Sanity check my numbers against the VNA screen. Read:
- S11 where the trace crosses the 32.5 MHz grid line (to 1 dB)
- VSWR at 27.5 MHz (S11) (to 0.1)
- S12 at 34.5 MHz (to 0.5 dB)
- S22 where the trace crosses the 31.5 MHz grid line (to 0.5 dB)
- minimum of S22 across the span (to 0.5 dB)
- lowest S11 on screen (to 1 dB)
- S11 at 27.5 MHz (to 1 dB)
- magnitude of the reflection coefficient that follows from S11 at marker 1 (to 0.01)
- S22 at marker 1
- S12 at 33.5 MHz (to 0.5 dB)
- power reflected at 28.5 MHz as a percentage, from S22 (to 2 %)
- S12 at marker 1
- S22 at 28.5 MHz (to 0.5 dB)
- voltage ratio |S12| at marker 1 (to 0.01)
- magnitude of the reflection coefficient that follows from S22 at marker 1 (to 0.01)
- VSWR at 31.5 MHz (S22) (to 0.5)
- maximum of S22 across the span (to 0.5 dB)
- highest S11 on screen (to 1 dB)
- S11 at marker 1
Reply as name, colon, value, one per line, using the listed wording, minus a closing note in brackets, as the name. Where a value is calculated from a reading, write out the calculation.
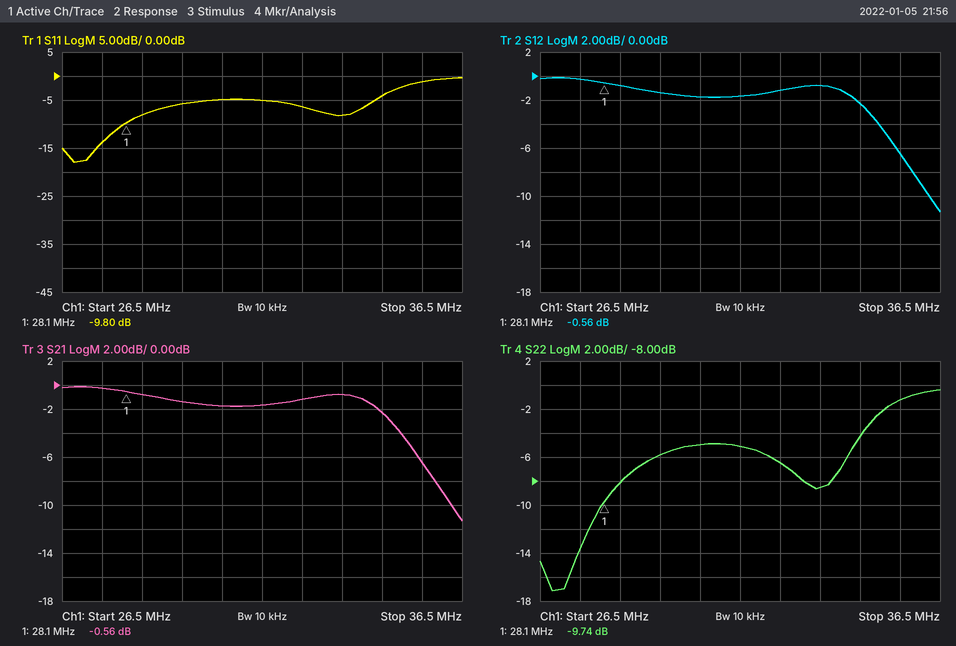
S11 where the trace crosses the 32.5 MHz grid line: -6 dB
VSWR at 27.5 MHz (S11): |Γ| = 10^(-14/20) = 0.1995; VSWR = (1 + 0.1995)/(1 − 0.1995) ≈ 1.5
S12 at 34.5 MHz: -2.5 dB
S22 where the trace crosses the 31.5 MHz grid line: -5.0 dB
minimum of S22 across the span: -17.0 dB
lowest S11 on screen: -18 dB
S11 at 27.5 MHz: -14 dB
magnitude of the reflection coefficient that follows from S11 at marker 1: 10^(-9.8/20) ≈ 0.32
S22 at marker 1: -9.74 dB
S12 at 33.5 MHz: -1.0 dB
power reflected at 28.5 MHz as a percentage, from S22: 10^(-8/10) ≈ 16 %
S12 at marker 1: -0.56 dB
S22 at 28.5 MHz: -8.0 dB
voltage ratio |S12| at marker 1: 10^(-0.56/20) ≈ 0.94
magnitude of the reflection coefficient that follows from S22 at marker 1: 10^(-9.74/20) ≈ 0.33
VSWR at 31.5 MHz (S22): |Γ| = 10^(-5/20) = 0.5623; VSWR = (1 + 0.5623)/(1 − 0.5623) ≈ 3.57, so 3.5 to the nearest 0.5
maximum of S22 across the span: -0.5 dB
highest S11 on screen: 0 dB
S11 at marker 1: -9.80 dB
